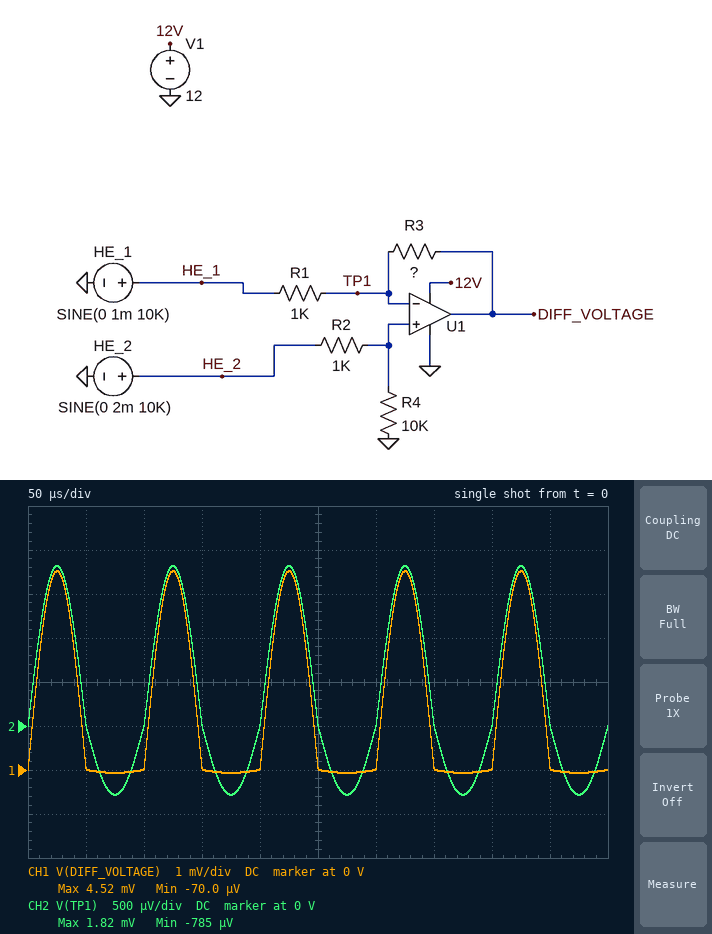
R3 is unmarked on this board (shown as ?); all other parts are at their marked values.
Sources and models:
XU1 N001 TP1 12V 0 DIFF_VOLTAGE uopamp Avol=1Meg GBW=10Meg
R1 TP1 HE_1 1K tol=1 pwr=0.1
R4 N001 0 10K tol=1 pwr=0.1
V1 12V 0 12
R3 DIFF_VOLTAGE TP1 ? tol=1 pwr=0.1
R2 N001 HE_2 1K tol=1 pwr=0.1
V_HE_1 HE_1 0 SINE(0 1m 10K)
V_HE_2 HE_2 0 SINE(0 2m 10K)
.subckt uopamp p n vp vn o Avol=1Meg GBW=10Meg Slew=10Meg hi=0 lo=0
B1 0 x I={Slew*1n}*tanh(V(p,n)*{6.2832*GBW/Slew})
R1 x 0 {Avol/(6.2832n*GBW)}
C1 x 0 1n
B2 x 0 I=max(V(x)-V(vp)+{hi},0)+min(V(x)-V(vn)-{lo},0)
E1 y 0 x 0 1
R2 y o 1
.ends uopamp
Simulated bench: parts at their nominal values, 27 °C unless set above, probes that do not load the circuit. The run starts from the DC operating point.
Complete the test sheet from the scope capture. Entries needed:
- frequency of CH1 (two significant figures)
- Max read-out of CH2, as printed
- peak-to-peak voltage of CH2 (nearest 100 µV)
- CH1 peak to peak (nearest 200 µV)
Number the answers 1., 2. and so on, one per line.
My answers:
1. 10 kHz
2. 1.82 mV
3. 2.6 mV
4. 4.6 mV
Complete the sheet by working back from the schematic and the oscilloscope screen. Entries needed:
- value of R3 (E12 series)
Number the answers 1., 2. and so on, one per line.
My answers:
1. 3.3 kΩ
